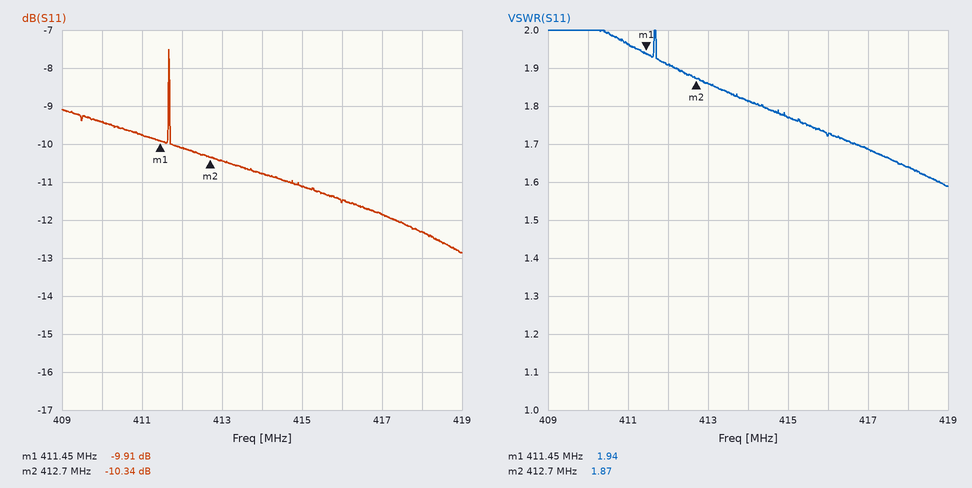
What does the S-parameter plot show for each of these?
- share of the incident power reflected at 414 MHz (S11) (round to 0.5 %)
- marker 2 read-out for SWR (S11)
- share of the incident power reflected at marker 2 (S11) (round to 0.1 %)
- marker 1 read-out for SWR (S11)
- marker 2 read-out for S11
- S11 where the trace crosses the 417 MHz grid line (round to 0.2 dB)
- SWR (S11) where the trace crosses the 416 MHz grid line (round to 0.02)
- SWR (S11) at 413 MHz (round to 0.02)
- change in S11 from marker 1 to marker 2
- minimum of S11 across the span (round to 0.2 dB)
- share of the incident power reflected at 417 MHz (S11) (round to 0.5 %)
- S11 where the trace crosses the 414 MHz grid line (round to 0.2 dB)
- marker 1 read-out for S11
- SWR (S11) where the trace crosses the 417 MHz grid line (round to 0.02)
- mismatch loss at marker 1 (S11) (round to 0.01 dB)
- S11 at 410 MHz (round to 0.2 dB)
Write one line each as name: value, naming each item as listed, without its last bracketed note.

share of the incident power reflected at 414 MHz (S11): 8.5 %
marker 2 read-out for SWR: 1.87
share of the incident power reflected at marker 2 (S11): 9.2 %
marker 1 read-out for SWR: 1.94
marker 2 read-out for S11: -10.34 dB
S11 where the trace crosses the 417 MHz grid line: -11.8 dB
SWR (S11) where the trace crosses the 416 MHz grid line: 1.72
SWR (S11) at 413 MHz: 1.86
change in S11 from marker 1 to marker 2: -0.43 dB
minimum of S11 across the span: -12.8 dB
share of the incident power reflected at 417 MHz (S11): 6.5 %
S11 where the trace crosses the 414 MHz grid line: -10.8 dB
marker 1 read-out for S11: -9.91 dB
SWR (S11) where the trace crosses the 417 MHz grid line: 1.68
mismatch loss at marker 1 (S11): 0.47 dB
S11 at 410 MHz: -9.4 dB
